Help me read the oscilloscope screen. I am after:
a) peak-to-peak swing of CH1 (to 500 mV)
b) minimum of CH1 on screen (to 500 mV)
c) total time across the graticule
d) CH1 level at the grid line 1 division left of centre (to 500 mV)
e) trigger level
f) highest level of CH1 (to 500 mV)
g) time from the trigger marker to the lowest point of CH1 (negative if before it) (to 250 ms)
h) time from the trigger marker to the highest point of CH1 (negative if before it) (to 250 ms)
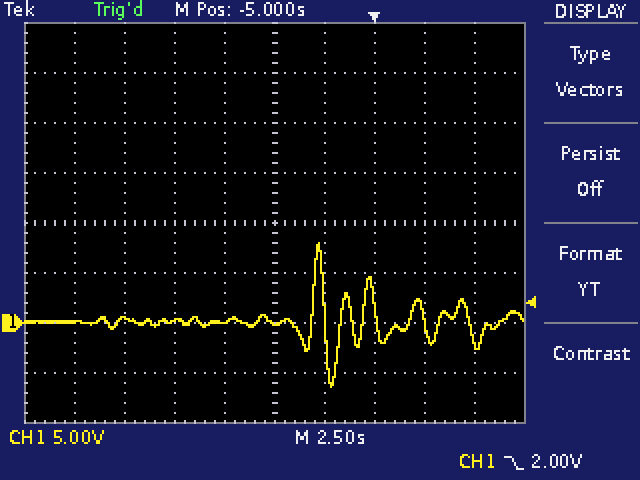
14.5 V
-6.5 V
25 s
0.0 V
2.00 V
8.0 V
-2.25 s
-2.75 s
